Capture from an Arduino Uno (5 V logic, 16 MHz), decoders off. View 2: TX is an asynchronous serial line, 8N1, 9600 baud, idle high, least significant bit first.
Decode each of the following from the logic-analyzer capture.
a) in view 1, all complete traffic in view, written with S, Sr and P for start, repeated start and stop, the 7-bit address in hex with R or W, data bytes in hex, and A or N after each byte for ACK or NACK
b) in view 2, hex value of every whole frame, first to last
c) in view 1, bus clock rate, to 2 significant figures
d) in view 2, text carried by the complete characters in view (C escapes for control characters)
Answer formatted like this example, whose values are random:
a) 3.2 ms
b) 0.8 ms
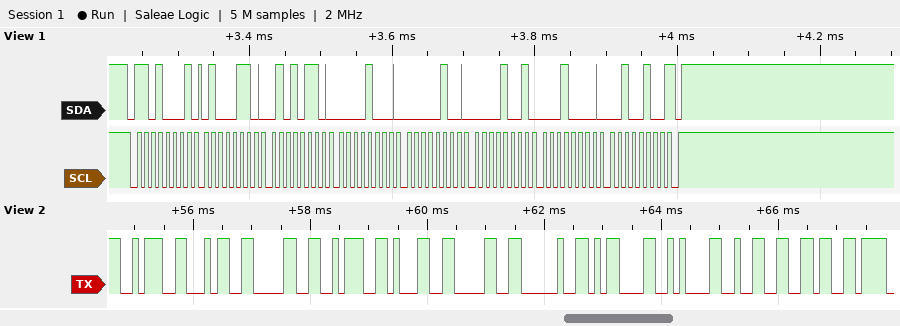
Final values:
a) S 68R A 46 A 56 A 08 A 04 A 09 A 10 A 24 N P
b) 0x3A 0x34 0x30 0x3A 0x31 0x30 0x20 0x0D 0x0A 0x32 0x36
c) 100 kHz
d) ":40:10 \r\n26"
